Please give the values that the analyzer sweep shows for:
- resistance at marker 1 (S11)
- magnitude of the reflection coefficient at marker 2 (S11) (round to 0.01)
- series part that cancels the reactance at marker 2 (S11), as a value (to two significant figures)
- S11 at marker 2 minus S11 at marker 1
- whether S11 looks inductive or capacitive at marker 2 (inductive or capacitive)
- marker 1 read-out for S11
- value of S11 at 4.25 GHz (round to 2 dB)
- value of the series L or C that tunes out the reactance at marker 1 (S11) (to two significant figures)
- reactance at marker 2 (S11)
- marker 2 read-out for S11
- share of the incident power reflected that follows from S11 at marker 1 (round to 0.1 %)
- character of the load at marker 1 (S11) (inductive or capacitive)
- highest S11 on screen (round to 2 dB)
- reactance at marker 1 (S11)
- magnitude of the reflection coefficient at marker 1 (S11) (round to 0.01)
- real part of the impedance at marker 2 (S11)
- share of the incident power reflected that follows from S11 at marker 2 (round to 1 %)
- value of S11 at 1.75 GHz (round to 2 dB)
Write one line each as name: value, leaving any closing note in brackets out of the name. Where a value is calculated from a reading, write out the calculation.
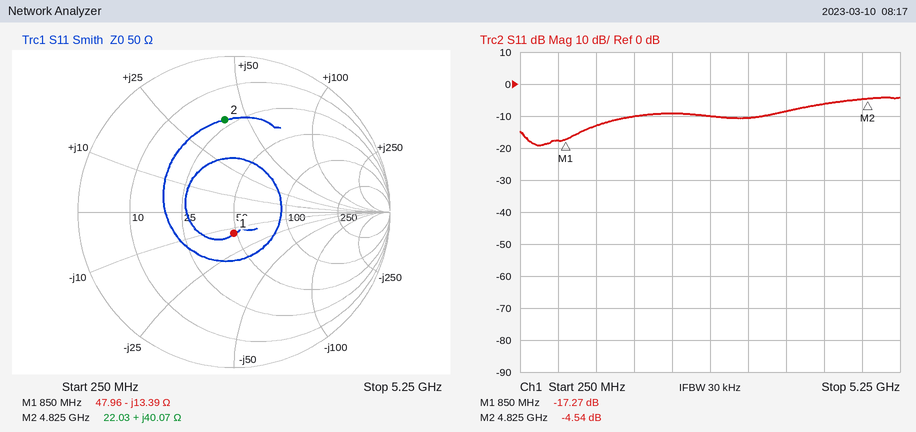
resistance at marker 1: 47.96 Ω
magnitude of the reflection coefficient at marker 2 (S11): 0.59
series part that cancels the reactance at marker 2 (S11), as a value: C = 1/(2π × 4.825 GHz × 40.07 Ω) ≈ 823 fF, so 820 fF to two significant figures
S11 at marker 2 minus S11 at marker 1: -4.54 − (-17.27) = 12.73 dB
whether S11 looks inductive or capacitive at marker 2: inductive
marker 1 read-out for S11: -17.27 dB
value of S11 at 4.25 GHz: -6 dB
value of the series L or C that tunes out the reactance at marker 1 (S11): L = 13.39 Ω/(2π × 850 MHz) ≈ 2.5 nH
reactance at marker 2: +40.07 Ω
marker 2 read-out for S11: -4.54 dB
share of the incident power reflected that follows from S11 at marker 1: 10^(-17.27/10) ≈ 1.9 %
character of the load at marker 1 (S11): capacitive
highest S11 on screen: -4 dB
reactance at marker 1: -13.39 Ω
magnitude of the reflection coefficient at marker 1 (S11): 0.14
real part of the impedance at marker 2: 22.03 Ω
share of the incident power reflected that follows from S11 at marker 2: 10^(-4.54/10) ≈ 35 %
value of S11 at 1.75 GHz: -10 dB
